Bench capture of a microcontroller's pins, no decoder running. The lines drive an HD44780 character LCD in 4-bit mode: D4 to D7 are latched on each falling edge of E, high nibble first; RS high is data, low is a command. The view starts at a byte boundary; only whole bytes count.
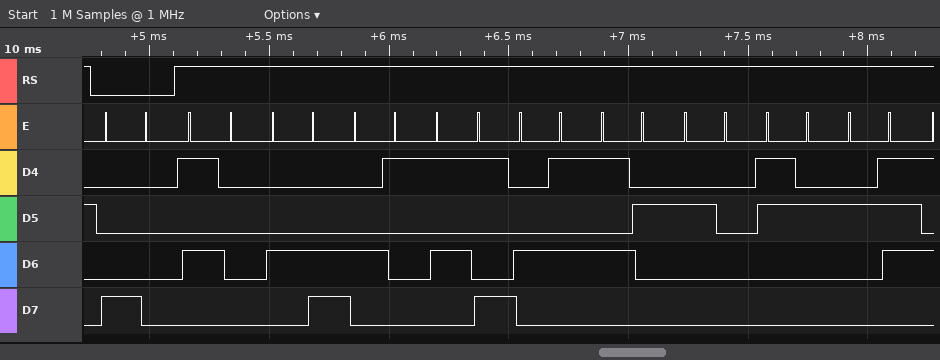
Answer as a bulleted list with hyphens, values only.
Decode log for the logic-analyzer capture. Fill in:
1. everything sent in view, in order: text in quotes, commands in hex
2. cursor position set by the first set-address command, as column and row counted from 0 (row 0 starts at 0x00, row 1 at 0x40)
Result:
- 0x80 "PLAYER 2'"
- column 0, row 0
